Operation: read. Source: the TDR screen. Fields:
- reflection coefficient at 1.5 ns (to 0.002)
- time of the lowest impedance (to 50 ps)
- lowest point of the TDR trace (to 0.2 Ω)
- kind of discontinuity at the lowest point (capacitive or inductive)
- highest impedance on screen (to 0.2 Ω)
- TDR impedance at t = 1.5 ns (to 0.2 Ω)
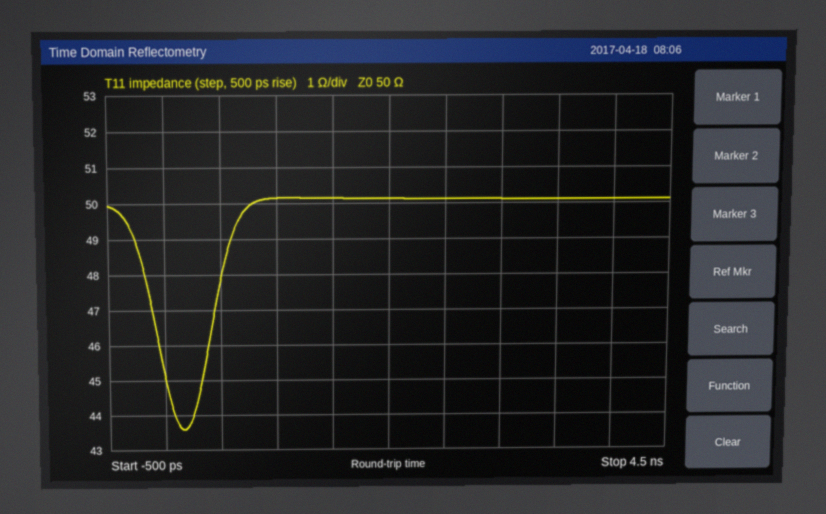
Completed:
+0.002
150 ps
43.6 Ω
capacitive
50.2 Ω
50.2 Ω
